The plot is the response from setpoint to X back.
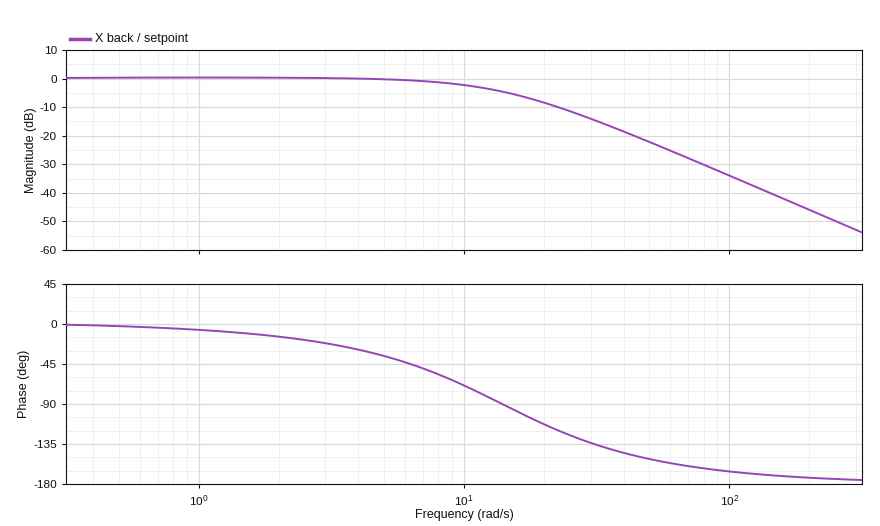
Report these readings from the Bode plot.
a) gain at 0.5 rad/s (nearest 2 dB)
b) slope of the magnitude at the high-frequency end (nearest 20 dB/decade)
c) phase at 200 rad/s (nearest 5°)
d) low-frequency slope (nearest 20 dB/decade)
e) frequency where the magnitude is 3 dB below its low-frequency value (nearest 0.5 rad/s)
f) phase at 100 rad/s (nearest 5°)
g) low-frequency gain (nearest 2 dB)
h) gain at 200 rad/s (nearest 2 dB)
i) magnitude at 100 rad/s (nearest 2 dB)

0 dB
-40 dB/decade
-175°
0 dB/decade
11.0 rad/s
-165°
0 dB
-46 dB
-34 dB
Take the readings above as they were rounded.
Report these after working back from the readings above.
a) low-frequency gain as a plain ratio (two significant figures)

1.0
